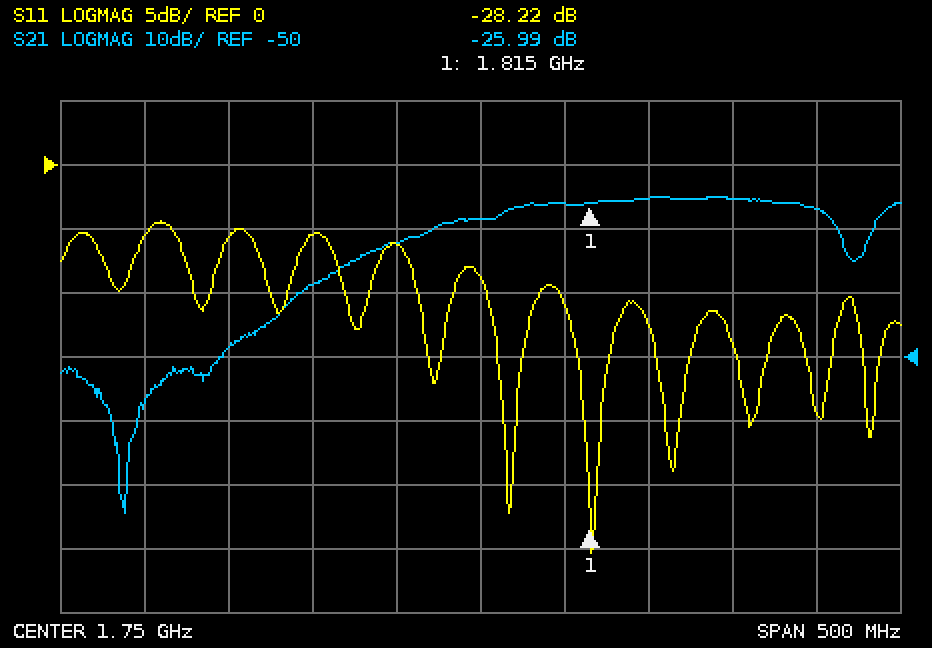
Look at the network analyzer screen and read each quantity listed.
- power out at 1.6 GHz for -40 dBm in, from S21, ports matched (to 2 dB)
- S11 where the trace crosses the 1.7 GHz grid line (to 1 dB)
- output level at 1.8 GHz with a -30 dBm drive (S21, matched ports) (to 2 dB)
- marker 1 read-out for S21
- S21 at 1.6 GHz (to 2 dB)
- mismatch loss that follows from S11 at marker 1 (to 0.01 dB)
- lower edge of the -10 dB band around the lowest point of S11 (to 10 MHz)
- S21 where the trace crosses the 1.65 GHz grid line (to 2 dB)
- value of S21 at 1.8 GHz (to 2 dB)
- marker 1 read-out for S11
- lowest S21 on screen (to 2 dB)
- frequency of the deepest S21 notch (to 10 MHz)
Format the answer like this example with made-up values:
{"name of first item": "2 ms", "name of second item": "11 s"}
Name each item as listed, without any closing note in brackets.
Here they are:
{"power out at 1.6 GHz for -40 dBm in, from S21, ports matched": "-88 dBm", "S11 where the trace crosses the 1.7 GHz grid line": "-6 dB", "output level at 1.8 GHz with a -30 dBm drive (S21, matched ports)": "-56 dBm", "marker 1 read-out for S21": "-25.99 dB", "S21 at 1.6 GHz": "-48 dB", "mismatch loss that follows from S11 at marker 1": "0.01 dB", "lower edge of the -10 dB band around the lowest point of S11": "1.80 GHz", "S21 where the trace crosses the 1.65 GHz grid line": "-38 dB", "value of S21 at 1.8 GHz": "-26 dB", "marker 1 read-out for S11": "-28.22 dB", "lowest S21 on screen": "-74 dB", "frequency of the deepest S21 notch": "1.54 GHz"}
